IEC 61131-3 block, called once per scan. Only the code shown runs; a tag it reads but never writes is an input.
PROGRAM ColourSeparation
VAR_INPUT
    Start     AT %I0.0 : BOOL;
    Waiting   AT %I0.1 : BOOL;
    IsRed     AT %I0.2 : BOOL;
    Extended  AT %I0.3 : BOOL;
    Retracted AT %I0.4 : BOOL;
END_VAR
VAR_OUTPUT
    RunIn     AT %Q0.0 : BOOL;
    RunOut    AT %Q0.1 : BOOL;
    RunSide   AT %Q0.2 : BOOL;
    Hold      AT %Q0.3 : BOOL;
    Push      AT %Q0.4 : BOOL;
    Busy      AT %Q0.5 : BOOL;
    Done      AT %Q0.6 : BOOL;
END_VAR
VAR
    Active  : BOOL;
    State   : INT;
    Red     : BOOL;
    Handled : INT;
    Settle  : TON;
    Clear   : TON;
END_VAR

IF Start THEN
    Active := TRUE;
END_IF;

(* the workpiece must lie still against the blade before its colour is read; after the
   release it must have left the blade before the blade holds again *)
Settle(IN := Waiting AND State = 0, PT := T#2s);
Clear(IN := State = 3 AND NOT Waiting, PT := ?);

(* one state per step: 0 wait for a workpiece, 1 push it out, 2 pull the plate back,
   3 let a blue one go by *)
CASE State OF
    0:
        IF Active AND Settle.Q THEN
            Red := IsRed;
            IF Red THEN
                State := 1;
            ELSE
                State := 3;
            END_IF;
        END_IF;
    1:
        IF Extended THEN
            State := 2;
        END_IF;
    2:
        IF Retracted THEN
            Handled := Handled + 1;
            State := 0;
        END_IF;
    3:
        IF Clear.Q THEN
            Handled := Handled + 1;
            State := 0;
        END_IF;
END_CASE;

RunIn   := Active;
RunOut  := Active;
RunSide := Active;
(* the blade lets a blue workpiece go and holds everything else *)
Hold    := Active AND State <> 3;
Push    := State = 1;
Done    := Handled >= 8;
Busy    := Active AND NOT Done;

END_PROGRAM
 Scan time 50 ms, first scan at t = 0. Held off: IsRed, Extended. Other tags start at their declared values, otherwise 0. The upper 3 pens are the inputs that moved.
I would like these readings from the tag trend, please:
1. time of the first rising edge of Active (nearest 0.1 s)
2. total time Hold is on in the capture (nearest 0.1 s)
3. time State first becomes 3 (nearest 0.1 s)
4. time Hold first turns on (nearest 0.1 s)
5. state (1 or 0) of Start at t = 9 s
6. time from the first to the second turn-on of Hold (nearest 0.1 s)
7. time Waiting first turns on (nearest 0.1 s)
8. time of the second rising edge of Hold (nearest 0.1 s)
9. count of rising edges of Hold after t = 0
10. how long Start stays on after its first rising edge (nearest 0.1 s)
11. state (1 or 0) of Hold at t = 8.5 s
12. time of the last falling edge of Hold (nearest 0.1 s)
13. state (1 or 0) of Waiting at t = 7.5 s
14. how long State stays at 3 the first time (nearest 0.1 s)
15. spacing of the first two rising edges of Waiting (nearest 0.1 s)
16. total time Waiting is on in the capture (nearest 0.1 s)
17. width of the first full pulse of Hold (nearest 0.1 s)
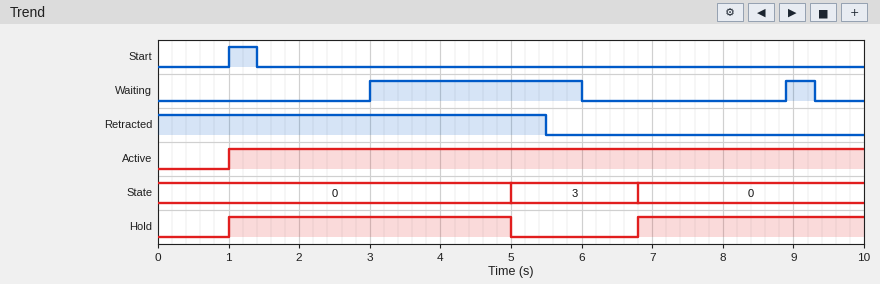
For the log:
1.0 s
7.2 s
5.0 s
1.0 s
0
5.8 s
3.0 s
6.8 s
2
0.4 s
1
5.0 s
0
1.8 s
5.9 s
3.4 s
4.0 s
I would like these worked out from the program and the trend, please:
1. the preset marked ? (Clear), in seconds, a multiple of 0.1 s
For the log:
0.8 s
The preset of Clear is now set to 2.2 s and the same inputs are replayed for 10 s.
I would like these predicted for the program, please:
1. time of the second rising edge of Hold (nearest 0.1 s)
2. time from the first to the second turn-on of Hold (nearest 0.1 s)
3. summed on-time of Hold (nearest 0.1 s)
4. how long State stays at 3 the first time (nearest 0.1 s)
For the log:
8.2 s
7.2 s
5.8 s
3.2 s
